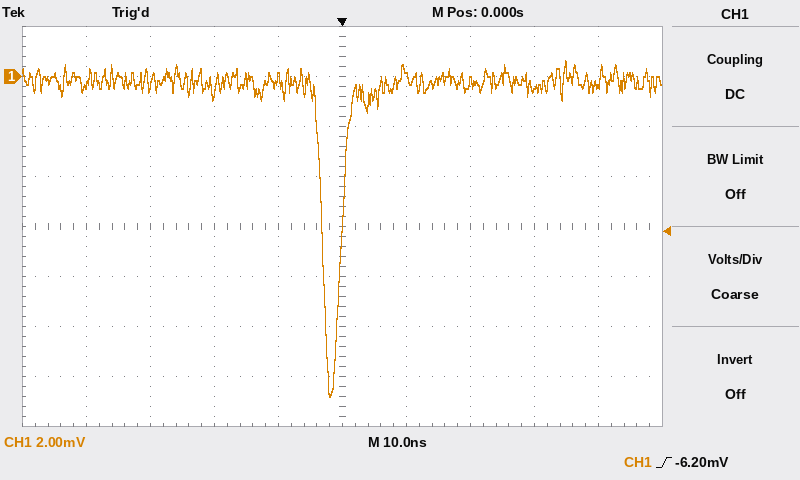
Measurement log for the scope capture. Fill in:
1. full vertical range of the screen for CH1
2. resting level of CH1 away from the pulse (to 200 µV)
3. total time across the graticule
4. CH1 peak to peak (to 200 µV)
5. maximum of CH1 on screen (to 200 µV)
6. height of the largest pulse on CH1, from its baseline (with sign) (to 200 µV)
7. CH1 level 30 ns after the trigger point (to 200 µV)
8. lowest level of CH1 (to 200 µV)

16 mV
-200 µV
100 ns
13.4 mV
600 µV
-12.6 mV
-400 µV
-12.8 mV
